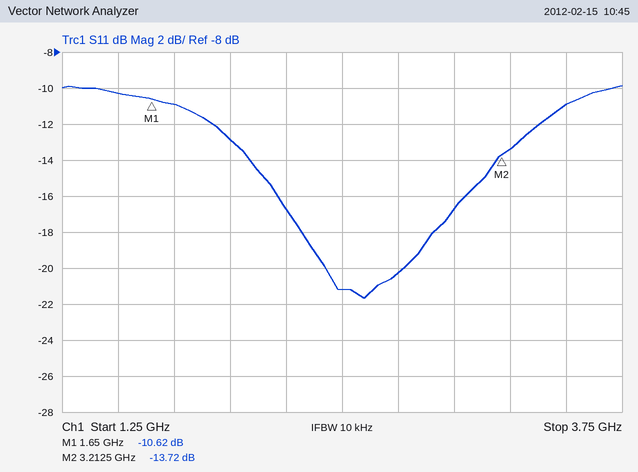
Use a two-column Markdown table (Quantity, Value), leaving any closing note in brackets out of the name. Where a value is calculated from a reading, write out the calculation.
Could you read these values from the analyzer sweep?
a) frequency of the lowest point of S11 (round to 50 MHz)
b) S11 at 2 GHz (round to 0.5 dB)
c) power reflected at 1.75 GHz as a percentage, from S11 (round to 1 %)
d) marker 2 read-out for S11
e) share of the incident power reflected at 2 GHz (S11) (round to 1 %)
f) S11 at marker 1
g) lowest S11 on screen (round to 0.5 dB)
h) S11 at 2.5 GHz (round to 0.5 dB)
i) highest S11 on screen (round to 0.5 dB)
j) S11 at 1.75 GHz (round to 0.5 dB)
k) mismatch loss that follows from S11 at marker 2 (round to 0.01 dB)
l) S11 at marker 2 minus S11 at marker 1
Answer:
| Quantity | Value |
|---|---|
| frequency of the lowest point of S11 | 2.60 GHz |
| S11 at 2 GHz | -13.0 dB |
| power reflected at 1.75 GHz as a percentage, from S11 | 10^(-11/10) ≈ 8 % |
| marker 2 read-out for S11 | -13.72 dB |
| share of the incident power reflected at 2 GHz (S11) | 10^(-13/10) ≈ 5 % |
| S11 at marker 1 | -10.62 dB |
| lowest S11 on screen | -21.5 dB |
| S11 at 2.5 GHz | -21.0 dB |
| highest S11 on screen | -10.0 dB |
| S11 at 1.75 GHz | -11.0 dB |
| mismatch loss that follows from S11 at marker 2 | −10 log10(1 − 10^(-13.72/10)) ≈ 0.19 dB |
| S11 at marker 2 minus S11 at marker 1 | -13.72 − (-10.62) = -3.10 dB |
